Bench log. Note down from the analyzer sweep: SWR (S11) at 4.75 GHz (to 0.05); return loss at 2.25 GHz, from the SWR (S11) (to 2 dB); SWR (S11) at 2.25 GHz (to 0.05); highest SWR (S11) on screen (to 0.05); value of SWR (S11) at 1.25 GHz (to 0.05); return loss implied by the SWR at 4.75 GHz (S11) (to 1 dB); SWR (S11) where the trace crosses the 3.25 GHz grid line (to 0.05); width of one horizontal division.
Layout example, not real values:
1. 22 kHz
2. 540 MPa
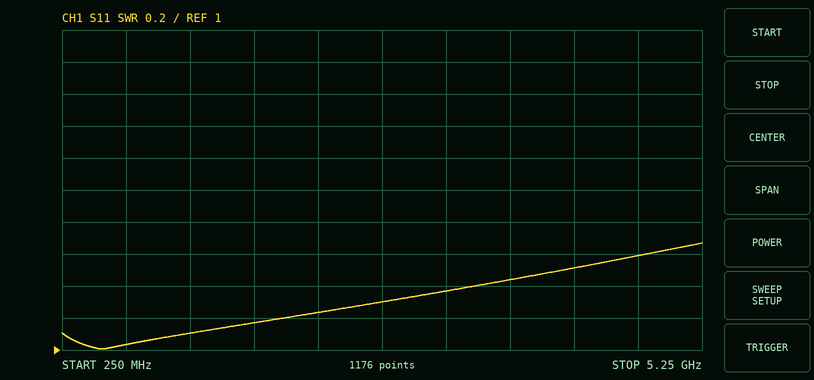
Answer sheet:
1. 1.60
2. 20 dB
3. 1.25
4. 1.65
5. 1.10
6. 13 dB
7. 1.35
8. 500 MHz
